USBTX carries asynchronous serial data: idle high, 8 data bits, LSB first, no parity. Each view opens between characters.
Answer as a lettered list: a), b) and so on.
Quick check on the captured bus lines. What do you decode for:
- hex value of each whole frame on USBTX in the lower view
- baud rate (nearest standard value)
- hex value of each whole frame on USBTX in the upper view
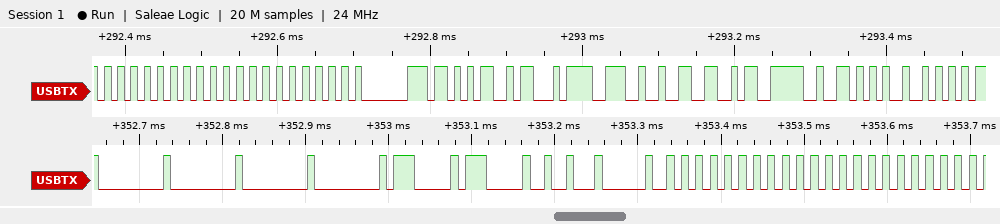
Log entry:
a) 00, 00, 00, 00, 07, 07, 12, 20, 55, 55, 55, 55
b) 115200 baud
c) 55, 55, 55, 55, C0, AB, 1A, CF, 92, A6, 3E, 56, 52
